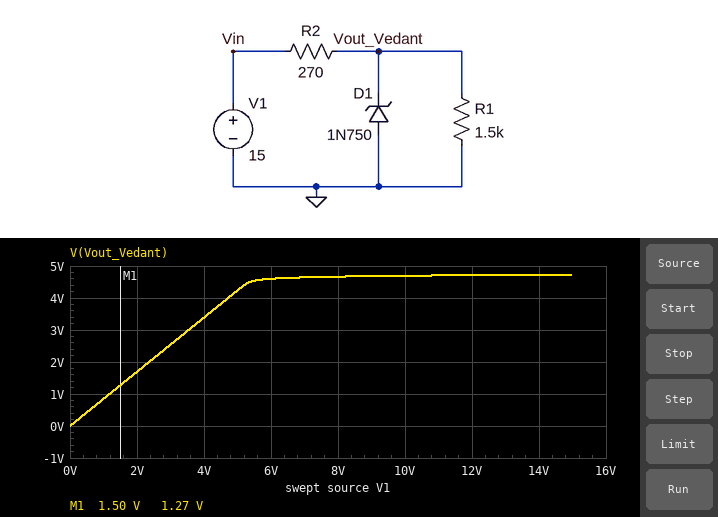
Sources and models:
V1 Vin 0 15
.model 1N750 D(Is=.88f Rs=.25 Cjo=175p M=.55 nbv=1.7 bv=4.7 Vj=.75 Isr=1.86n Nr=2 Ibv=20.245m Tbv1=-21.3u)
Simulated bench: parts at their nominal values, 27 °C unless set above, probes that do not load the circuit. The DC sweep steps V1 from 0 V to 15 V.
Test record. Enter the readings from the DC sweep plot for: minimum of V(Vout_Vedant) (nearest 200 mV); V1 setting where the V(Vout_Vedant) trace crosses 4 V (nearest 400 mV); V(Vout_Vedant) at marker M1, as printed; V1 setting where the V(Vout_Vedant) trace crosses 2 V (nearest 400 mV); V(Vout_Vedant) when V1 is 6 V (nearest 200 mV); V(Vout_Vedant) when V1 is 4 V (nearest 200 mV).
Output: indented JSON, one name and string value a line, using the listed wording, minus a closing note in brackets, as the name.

{
  "minimum of V(Vout_Vedant)": "0 V",
  "V1 setting where the V(Vout_Vedant) trace crosses 4 V": "4.8 V",
  "V(Vout_Vedant) at marker M1, as printed": "1.27 V",
  "V1 setting where the V(Vout_Vedant) trace crosses 2 V": "2.4 V",
  "V(Vout_Vedant) when V1 is 6 V": "4.6 V",
  "V(Vout_Vedant) when V1 is 4 V": "3.4 V"
}
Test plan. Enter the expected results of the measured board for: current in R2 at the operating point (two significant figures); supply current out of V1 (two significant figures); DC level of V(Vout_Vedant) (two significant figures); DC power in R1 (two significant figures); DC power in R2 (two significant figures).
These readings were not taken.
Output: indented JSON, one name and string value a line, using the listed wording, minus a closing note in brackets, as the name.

{
  "current in R2 at the operating point": "38 mA",
  "supply current out of V1": "38 mA",
  "DC level of V(Vout_Vedant)": "4.7 V",
  "DC power in R1": "15 mW",
  "DC power in R2": "390 mW"
}
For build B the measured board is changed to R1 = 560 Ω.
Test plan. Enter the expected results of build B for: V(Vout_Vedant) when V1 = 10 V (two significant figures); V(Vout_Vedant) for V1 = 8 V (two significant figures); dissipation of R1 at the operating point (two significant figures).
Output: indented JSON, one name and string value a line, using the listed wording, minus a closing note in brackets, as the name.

{
  "V(Vout_Vedant) when V1 = 10 V": "4.7 V",
  "V(Vout_Vedant) for V1 = 8 V": "4.6 V",
  "dissipation of R1 at the operating point": "40 mW"
}
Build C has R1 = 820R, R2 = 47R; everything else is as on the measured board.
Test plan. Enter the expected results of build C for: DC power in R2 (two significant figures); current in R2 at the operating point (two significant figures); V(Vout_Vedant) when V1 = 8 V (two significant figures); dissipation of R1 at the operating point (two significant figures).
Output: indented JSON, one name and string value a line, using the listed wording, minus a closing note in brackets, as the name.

{
  "DC power in R2": "2.2 W",
  "current in R2 at the operating point": "220 mA",
  "V(Vout_Vedant) when V1 = 8 V": "4.8 V",
  "dissipation of R1 at the operating point": "29 mW"
}
